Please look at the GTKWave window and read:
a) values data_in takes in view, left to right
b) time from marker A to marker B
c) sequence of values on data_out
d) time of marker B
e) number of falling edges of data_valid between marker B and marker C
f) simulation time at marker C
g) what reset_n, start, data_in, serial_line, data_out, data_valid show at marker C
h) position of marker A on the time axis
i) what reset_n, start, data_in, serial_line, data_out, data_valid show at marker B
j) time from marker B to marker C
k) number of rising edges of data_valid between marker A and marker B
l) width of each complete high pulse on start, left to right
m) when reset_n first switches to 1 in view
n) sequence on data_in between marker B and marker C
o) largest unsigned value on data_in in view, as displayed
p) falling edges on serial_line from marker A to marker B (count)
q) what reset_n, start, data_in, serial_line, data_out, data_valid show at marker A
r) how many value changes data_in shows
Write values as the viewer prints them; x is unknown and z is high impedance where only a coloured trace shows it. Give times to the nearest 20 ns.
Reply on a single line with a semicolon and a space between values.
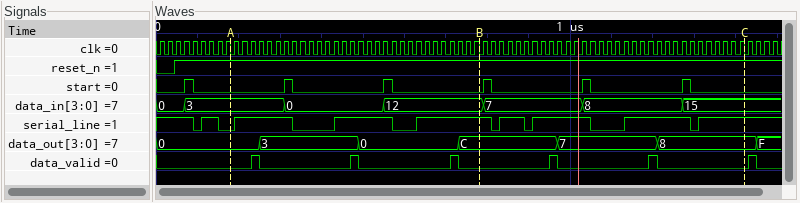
0, 3, 0, 12, 7, 8, 15; 600 ns; 0, 3, 0, C, 7, 8, F; 780 ns; 2; 1420 ns; reset_n=1, start=0, data_in=15, serial_line=1, data_out=8, data_valid=0; 180 ns; reset_n=1, start=0, data_in=12, serial_line=1, data_out=C, data_valid=0; 640 ns; 3; 20 ns, 20 ns, 20 ns, 20 ns, 20 ns, 20 ns; 40 ns; 12, 7, 8, 15; 15; 2; reset_n=1, start=0, data_in=3, serial_line=0, data_out=0, data_valid=0; 6
